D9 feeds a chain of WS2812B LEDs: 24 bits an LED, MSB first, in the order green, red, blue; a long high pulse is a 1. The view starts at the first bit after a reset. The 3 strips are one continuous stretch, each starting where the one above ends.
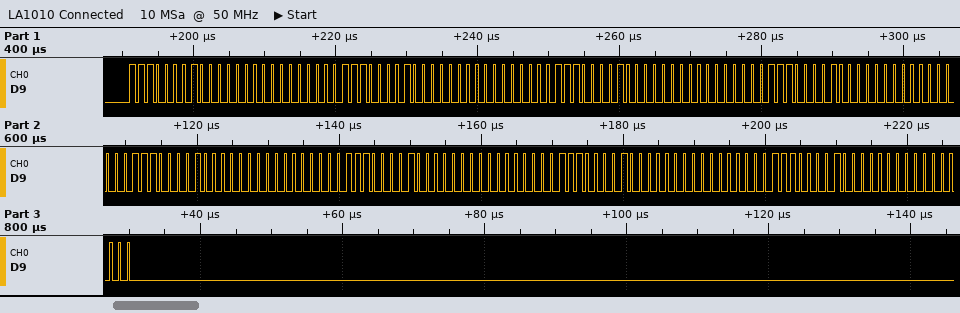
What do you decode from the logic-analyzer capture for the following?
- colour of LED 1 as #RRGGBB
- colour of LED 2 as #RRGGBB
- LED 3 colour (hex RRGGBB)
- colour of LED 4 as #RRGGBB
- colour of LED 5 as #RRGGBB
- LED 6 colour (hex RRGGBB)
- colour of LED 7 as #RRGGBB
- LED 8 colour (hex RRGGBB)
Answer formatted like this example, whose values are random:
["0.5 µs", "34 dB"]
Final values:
["#00E100", "#00E100", "#00E100", "#00E100", "#00E100", "#00E100", "#00E100", "#00E100"]
